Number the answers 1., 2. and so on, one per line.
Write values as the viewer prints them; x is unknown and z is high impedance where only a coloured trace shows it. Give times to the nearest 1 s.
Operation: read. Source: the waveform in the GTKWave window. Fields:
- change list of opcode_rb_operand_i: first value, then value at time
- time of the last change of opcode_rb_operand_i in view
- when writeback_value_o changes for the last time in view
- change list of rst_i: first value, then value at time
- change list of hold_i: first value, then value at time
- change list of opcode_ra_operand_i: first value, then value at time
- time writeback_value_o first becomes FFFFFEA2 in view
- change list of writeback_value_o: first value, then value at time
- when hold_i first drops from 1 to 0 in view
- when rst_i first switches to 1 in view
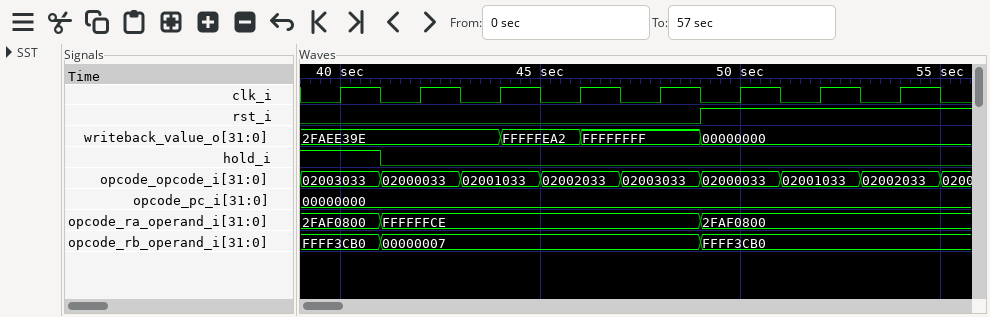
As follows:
1. FFFF3CB0, 00000007 at 41 s, FFFF3CB0 at 49 s
2. 49 s
3. 49 s
4. 0, 1 at 49 s
5. 1, 0 at 41 s
6. 2FAF0800, FFFFFFCE at 41 s, 2FAF0800 at 49 s
7. 44 s
8. 2FAEE39E, FFFFFEA2 at 44 s, FFFFFFFF at 46 s, 00000000 at 49 s
9. 41 s
10. 49 s
